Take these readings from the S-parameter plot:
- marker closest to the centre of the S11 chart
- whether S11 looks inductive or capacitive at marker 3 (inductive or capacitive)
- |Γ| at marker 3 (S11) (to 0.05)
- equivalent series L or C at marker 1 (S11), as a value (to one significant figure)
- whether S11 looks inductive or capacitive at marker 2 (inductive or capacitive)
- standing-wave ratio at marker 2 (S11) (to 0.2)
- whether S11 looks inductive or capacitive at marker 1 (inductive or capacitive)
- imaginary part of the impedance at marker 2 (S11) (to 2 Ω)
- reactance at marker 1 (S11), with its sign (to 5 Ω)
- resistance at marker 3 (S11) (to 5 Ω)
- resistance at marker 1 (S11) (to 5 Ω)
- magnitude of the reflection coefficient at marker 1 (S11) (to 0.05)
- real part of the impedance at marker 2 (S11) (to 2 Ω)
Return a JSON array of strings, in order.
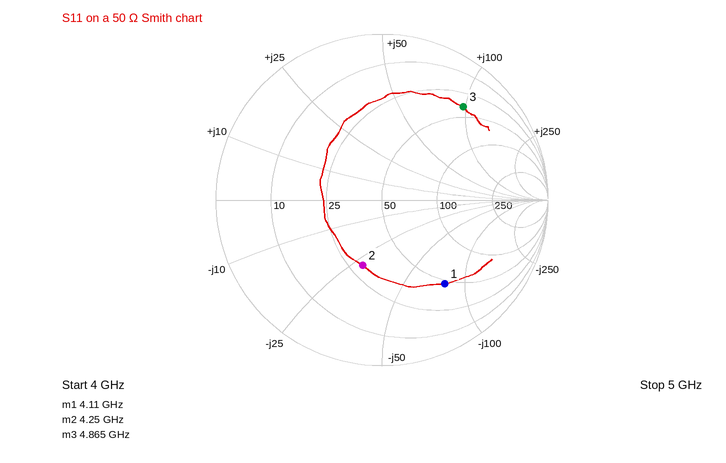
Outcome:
["marker 2", "inductive", "0.75", "500 fF", "capacitive", "2.4", "capacitive", "-28 Ω", "-80 Ω", "40 Ω", "45 Ω", "0.65", "30 Ω"]
